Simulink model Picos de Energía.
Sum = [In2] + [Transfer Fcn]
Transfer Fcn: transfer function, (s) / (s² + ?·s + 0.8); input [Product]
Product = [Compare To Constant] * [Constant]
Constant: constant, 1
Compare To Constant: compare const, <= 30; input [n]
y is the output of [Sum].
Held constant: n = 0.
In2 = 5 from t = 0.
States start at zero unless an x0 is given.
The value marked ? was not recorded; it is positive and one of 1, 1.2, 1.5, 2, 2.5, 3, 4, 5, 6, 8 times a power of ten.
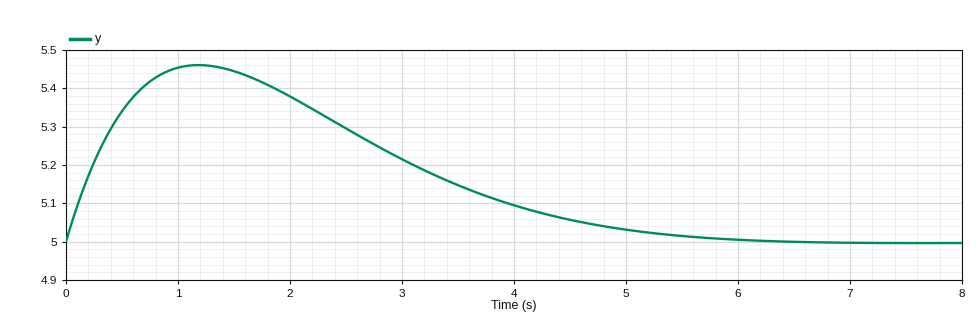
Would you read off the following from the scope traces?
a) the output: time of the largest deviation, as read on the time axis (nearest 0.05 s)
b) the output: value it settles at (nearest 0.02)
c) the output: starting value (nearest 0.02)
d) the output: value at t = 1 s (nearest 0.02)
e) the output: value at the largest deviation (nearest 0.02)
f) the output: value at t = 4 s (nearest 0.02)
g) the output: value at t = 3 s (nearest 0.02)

1.20 s
5.00
5.00
5.46
5.46
5.10
5.22
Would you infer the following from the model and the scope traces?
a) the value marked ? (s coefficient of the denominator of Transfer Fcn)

1.5
